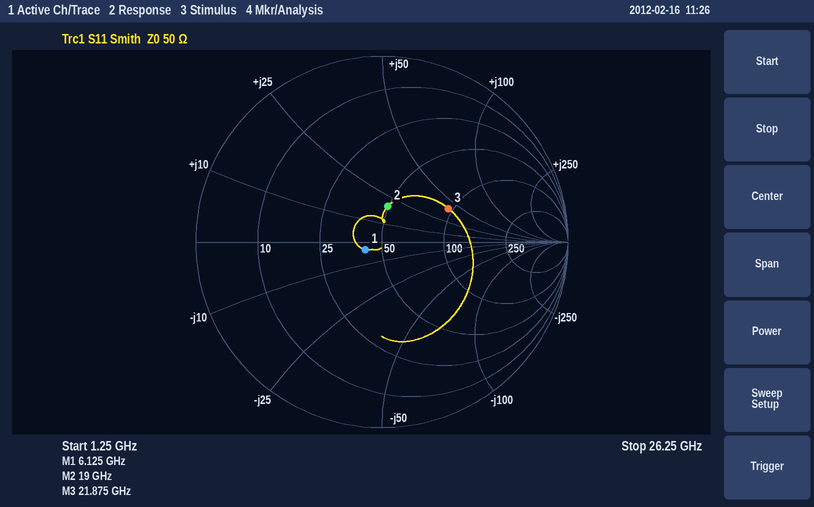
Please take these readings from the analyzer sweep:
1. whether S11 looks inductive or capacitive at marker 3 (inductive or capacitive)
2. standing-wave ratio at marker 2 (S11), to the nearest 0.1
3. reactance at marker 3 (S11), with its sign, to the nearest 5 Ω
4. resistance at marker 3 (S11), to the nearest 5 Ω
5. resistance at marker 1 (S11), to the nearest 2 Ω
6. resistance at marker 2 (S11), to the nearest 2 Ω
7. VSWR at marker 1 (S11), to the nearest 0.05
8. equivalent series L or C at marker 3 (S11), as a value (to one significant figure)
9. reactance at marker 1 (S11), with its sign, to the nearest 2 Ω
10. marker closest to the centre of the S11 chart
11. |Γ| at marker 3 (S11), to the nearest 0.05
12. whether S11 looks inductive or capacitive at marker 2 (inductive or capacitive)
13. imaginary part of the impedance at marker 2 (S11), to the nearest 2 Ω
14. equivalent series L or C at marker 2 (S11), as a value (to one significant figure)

inductive
1.5
+40 Ω
95 Ω
42 Ω
50 Ω
1.20
300 pH
-4 Ω
marker 1
0.40
inductive
+20 Ω
200 pH
